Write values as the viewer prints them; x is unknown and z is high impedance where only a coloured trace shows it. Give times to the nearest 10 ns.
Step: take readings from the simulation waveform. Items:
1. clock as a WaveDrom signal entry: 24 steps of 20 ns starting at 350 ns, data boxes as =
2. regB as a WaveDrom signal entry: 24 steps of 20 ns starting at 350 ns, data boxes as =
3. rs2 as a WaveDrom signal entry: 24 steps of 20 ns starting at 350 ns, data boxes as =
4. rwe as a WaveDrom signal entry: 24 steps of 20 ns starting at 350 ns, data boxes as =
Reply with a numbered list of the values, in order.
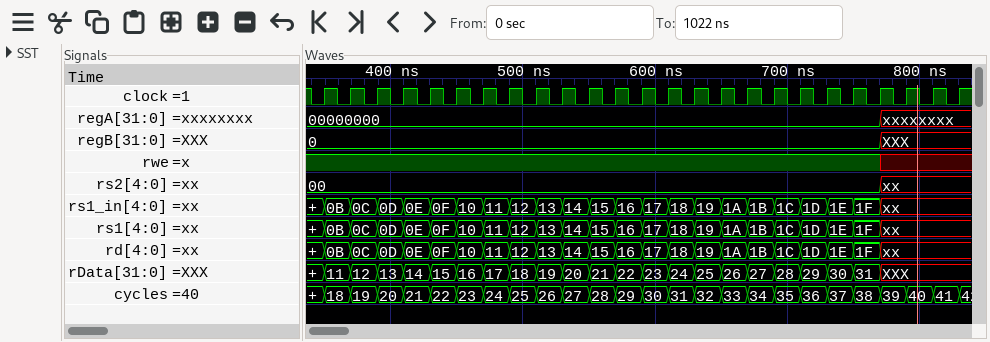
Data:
1. {name: 'clock', wave: 'p.......................'}
2. {name: 'regB', wave: '=....................x..', data: '0'}
3. {name: 'rs2', wave: '=....................x..', data: '00'}
4. {name: 'rwe', wave: '1....................x..'}
